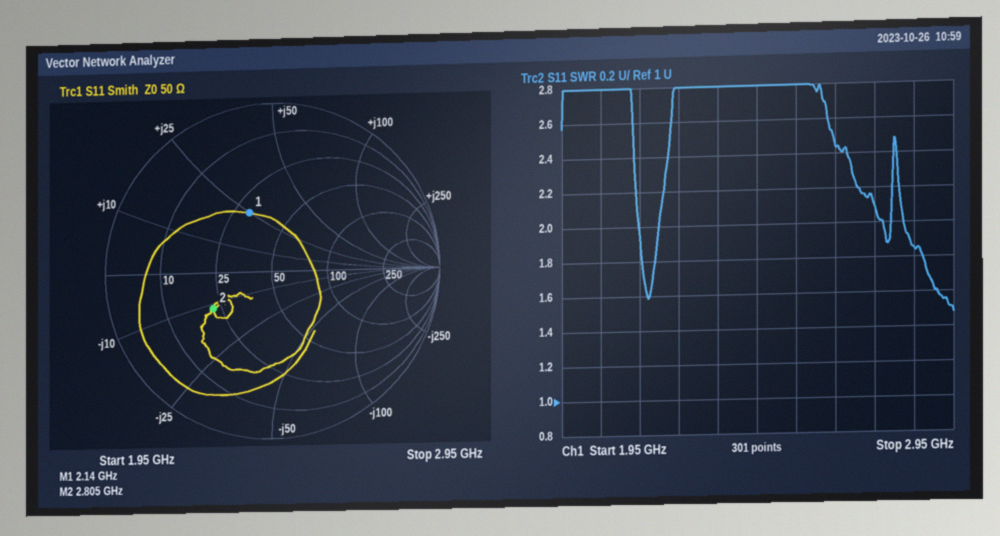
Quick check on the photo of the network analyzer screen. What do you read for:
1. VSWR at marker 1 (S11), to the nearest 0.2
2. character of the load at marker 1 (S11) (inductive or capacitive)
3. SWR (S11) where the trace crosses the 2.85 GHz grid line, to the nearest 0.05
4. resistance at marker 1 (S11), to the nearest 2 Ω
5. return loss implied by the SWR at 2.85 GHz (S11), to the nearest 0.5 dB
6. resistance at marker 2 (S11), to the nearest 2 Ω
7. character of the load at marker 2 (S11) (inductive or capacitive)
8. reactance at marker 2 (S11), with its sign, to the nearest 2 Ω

2.2
inductive
1.85
30 Ω
10.5 dB
22 Ω
capacitive
-12 Ω
